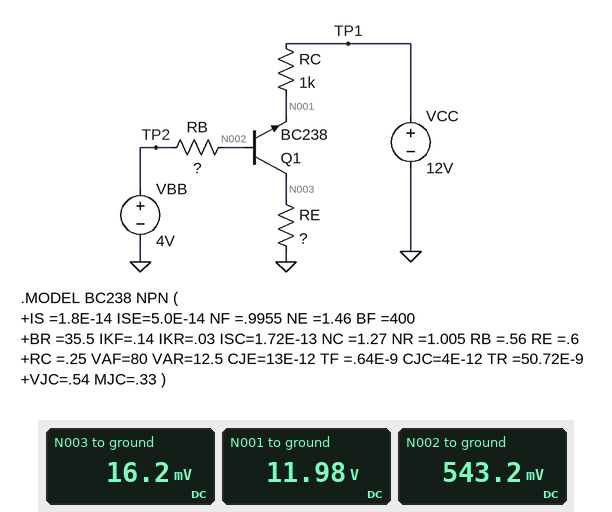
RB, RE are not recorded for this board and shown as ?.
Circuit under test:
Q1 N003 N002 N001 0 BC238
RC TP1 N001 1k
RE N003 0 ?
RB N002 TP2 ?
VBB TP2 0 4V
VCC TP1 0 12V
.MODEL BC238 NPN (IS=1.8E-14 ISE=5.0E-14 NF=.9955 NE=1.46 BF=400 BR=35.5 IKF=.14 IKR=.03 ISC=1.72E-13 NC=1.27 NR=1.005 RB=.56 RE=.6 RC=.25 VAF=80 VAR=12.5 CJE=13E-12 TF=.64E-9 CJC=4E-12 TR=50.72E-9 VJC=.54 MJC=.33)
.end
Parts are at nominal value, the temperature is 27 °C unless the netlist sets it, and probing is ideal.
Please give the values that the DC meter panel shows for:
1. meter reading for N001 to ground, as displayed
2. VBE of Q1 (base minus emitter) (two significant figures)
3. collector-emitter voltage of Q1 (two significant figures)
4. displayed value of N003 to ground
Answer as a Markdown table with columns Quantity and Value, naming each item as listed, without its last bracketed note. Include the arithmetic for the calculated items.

| Quantity | Value |
|---|---|
| meter reading for N001 to ground, as displayed | 11.98 V |
| VBE of Q1 (base minus emitter) | 543.2 mV - 11.98 V = -11 V |
| collector-emitter voltage of Q1 | 16.2 mV - 11.98 V = -12 V |
| displayed value of N003 to ground | 16.2 mV |
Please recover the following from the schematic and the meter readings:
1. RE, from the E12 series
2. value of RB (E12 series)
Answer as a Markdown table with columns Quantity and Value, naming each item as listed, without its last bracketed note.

| Quantity | Value |
|---|---|
| RE, from the E12 series | 680 Ω |
| value of RB | 1.8 MΩ |
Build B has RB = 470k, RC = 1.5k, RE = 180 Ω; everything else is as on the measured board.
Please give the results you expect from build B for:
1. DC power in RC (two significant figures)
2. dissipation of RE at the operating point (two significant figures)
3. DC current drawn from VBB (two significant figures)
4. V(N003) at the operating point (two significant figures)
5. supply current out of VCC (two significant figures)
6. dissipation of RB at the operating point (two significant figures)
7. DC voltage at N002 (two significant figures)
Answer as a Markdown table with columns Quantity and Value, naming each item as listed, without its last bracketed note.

| Quantity | Value |
|---|---|
| DC power in RC | 17 µW |
| dissipation of RE at the operating point | 2.4 µW |
| DC current drawn from VBB | 7.3 µA |
| V(N003) at the operating point | 21 mV |
| supply current out of VCC | 110 µA |
| dissipation of RB at the operating point | 25 µW |
| DC voltage at N002 | 590 mV |
